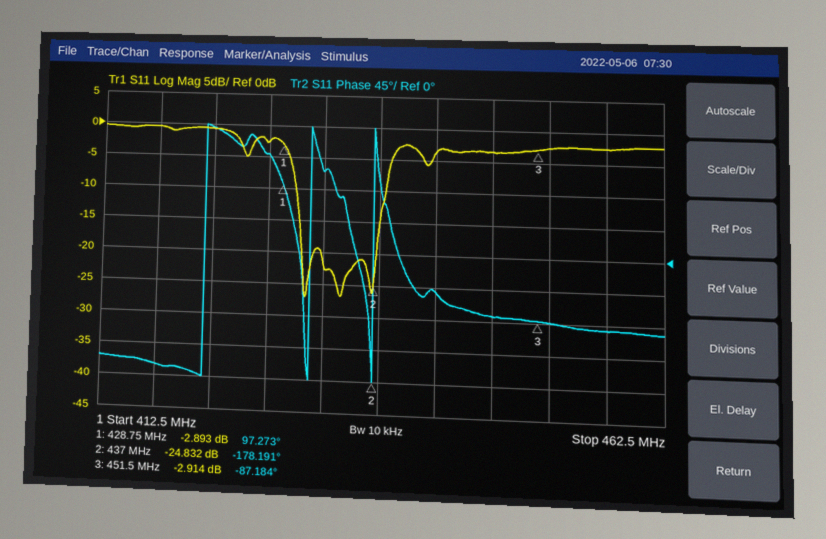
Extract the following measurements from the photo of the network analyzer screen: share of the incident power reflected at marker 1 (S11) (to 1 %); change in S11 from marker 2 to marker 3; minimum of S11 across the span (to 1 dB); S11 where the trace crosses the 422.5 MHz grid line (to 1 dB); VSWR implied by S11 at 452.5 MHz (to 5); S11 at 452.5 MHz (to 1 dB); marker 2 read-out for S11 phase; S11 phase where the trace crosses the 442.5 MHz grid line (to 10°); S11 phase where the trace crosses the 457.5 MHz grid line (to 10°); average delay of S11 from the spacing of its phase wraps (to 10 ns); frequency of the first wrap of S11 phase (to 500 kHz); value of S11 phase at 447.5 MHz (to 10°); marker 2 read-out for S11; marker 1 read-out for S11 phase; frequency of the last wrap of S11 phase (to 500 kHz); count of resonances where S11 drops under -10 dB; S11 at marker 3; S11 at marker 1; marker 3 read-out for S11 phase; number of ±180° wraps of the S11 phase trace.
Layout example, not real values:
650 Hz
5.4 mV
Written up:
51 %
21.918 dB
-27 dB
-1 dB
5
-3 dB
-178.191°
-50°
-100°
130 ns
422.0 MHz
-80°
-24.832 dB
97.273°
437.0 MHz
3
-2.914 dB
-2.893 dB
-87.184°
3
